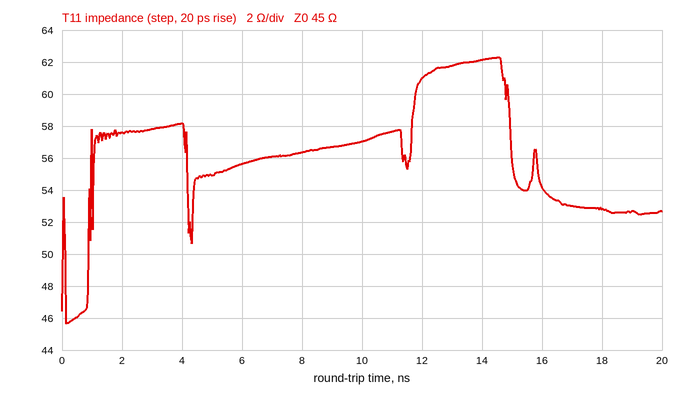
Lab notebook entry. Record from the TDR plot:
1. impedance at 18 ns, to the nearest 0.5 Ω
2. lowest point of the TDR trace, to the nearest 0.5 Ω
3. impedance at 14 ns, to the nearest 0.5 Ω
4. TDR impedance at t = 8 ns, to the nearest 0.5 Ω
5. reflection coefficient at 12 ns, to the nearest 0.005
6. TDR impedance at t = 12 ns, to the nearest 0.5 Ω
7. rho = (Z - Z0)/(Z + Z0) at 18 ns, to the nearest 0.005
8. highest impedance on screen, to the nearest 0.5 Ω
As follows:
53.0 Ω
45.5 Ω
62.0 Ω
56.5 Ω
+0.150
61.0 Ω
+0.080
62.5 Ω
